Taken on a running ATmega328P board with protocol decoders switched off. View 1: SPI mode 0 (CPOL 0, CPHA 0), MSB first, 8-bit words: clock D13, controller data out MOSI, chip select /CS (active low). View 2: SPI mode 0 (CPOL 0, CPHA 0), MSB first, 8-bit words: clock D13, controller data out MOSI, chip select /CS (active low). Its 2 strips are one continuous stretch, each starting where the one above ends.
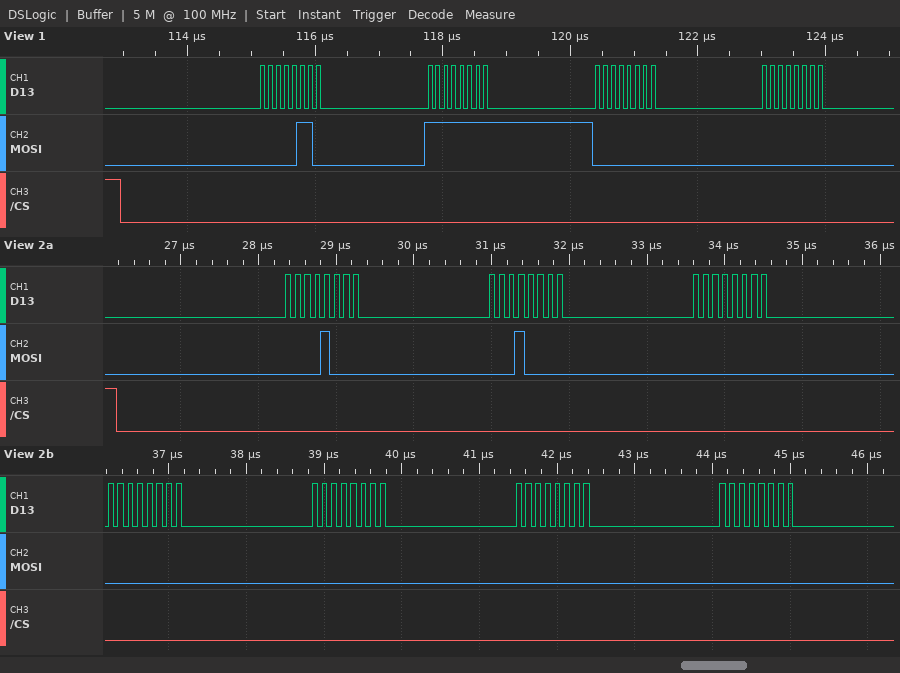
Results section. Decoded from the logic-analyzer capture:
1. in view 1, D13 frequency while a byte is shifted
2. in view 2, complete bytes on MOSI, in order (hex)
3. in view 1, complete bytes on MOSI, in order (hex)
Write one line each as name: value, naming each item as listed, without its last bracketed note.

in view 1, D13 frequency while a byte is shifted: 8 MHz
in view 2, complete bytes on MOSI, in order: 08 10 00 00 00 00 00
in view 1, complete bytes on MOSI, in order: 06 FF 00 00
